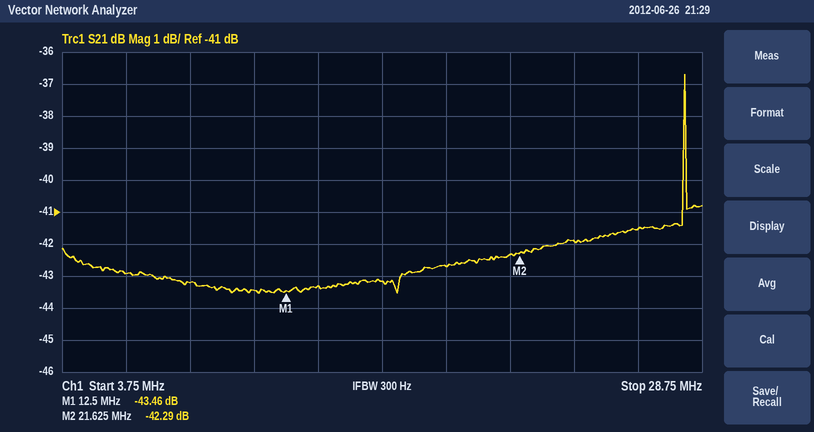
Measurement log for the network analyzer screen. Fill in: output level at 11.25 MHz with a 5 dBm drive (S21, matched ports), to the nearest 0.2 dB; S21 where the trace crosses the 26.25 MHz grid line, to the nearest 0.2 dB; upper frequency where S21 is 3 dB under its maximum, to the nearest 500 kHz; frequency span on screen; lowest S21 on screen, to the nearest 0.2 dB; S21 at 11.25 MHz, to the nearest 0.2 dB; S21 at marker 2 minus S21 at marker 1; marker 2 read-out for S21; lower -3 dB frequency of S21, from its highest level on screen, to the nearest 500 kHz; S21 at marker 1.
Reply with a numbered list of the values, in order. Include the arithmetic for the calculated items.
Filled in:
1. 5 dBm + (-43.4 dB) = -38.4 dBm
2. -41.6 dB
3. 28.0 MHz
4. 25 MHz
5. -43.6 dB
6. -43.4 dB
7. -42.29 − (-43.46) = 1.17 dB
8. -42.29 dB
9. 28.0 MHz
10. -43.46 dB
